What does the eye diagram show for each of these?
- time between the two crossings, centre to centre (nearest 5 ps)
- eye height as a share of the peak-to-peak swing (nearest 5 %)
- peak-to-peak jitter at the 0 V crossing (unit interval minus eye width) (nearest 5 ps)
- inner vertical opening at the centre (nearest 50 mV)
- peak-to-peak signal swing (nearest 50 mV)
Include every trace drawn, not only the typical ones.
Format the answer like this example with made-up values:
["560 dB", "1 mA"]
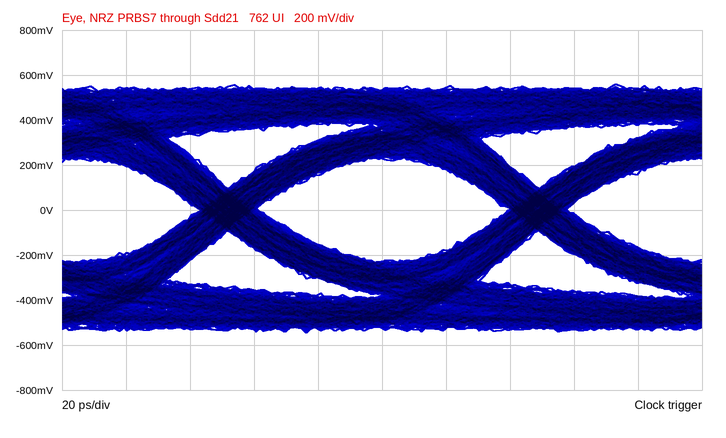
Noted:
["95 ps", "40 %", "20 ps", "450 mV", "1.10 V"]
